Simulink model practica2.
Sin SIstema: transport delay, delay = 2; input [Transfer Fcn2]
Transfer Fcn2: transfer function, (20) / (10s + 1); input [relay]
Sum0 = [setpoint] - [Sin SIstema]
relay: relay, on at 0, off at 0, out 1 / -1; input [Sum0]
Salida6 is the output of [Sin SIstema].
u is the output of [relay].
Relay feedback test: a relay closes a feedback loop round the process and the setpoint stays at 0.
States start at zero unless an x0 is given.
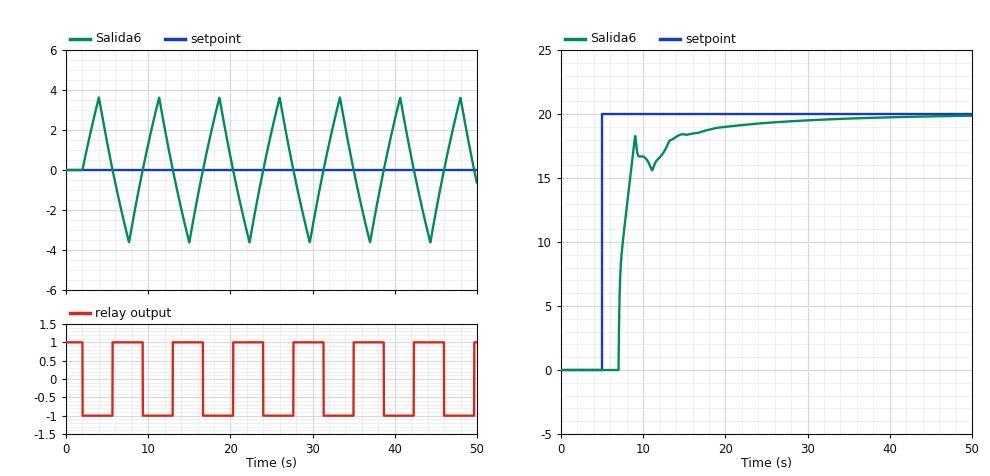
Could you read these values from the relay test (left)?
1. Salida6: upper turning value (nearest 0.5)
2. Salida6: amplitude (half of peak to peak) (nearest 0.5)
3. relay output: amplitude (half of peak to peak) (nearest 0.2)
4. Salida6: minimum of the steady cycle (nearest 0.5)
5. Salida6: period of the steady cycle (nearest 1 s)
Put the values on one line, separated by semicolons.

3.5; 3.5; 1.0; -3.5; 7 s
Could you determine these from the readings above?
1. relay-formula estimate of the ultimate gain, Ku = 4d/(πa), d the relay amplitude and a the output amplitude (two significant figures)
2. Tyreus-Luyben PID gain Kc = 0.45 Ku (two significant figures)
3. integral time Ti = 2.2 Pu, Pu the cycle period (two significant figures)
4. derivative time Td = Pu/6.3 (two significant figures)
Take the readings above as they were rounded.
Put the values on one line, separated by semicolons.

0.36; 0.16; 15 s; 1.1 s
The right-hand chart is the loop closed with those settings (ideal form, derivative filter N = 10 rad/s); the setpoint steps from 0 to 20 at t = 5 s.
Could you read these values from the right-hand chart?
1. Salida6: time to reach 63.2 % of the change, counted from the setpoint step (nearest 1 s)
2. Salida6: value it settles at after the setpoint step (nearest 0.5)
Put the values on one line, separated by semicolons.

3 s; 20.0
